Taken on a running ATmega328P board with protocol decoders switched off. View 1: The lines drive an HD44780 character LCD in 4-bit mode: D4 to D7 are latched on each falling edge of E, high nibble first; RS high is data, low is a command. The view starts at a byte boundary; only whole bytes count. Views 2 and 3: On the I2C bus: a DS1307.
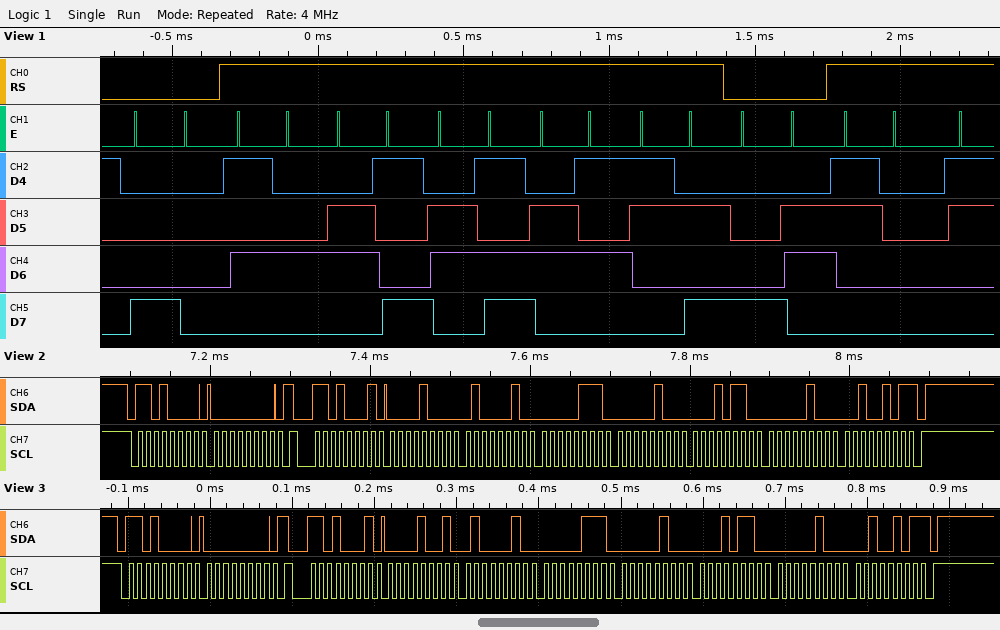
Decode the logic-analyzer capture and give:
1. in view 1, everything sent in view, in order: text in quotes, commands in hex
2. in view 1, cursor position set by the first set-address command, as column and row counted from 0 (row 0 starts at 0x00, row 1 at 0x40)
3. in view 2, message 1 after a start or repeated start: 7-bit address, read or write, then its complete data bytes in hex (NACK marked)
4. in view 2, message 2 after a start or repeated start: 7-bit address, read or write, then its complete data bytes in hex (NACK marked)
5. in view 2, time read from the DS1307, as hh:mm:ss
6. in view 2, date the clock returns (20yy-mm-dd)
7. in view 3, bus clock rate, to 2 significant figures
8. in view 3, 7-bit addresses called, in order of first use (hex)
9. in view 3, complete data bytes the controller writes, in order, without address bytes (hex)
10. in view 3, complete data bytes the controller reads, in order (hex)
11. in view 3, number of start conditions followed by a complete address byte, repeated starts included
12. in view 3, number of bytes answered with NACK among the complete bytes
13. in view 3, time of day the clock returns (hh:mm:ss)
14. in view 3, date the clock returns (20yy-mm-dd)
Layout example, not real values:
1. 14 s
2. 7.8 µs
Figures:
1. 0x80 "Time:" 0x86 "0"
2. column 0, row 0
3. 0x68 write: 00
4. 0x68 read: 08 42 07 04 16 04 25 NACK
5. 07:42:08
6. 2025-04-16
7. 100 kHz
8. 0x68
9. 00
10. 09 42 07 04 16 04 25
11. 2
12. 1
13. 07:42:09
14. 2025-04-16
